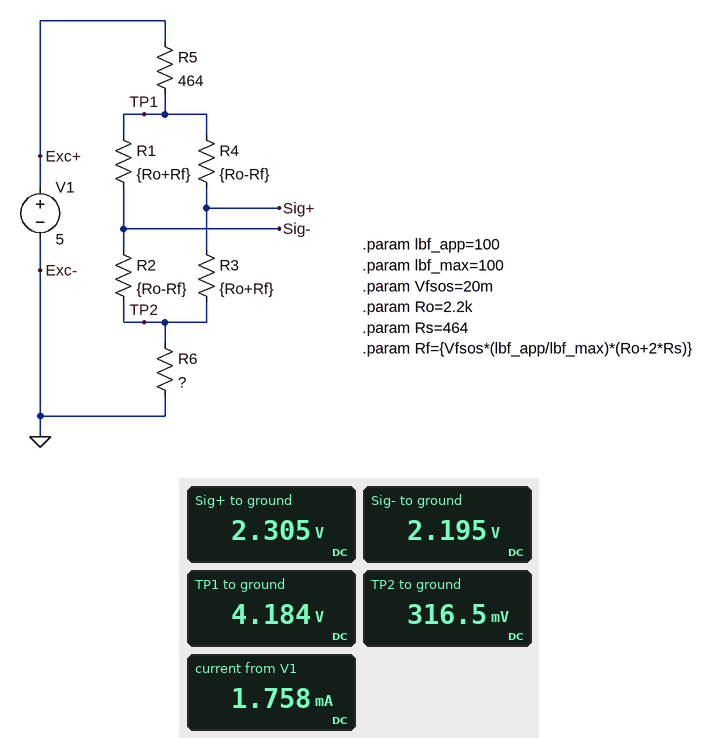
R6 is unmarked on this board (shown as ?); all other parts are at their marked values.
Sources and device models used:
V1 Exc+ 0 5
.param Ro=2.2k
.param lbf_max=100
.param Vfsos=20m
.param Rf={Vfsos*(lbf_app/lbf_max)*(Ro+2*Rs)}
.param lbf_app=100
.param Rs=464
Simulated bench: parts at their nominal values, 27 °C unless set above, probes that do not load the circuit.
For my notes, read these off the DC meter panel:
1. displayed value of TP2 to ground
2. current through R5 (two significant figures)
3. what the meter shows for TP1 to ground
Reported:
316.5 mV
1.8 mA
4.184 V
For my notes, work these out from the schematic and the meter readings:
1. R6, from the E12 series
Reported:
180 Ω
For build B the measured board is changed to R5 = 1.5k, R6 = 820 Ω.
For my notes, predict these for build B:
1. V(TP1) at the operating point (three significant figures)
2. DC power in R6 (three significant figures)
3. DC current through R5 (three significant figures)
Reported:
3.34 V
1.00 mW
1.11 mA
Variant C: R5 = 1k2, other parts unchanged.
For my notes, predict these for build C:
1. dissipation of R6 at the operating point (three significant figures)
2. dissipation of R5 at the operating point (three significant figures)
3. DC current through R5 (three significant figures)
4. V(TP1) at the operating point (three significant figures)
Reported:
351 µW
2.34 mW
1.40 mA
3.32 V
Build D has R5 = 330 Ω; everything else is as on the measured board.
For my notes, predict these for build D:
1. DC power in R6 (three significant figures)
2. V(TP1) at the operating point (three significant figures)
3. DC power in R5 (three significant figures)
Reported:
613 µW
4.39 V
1.12 mW
